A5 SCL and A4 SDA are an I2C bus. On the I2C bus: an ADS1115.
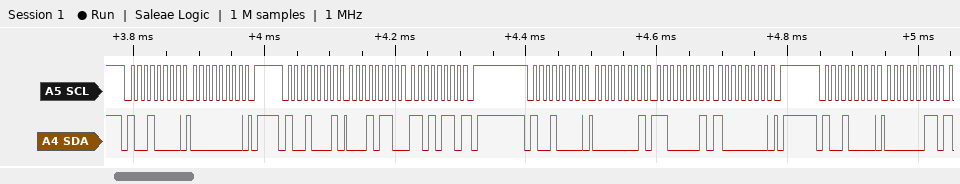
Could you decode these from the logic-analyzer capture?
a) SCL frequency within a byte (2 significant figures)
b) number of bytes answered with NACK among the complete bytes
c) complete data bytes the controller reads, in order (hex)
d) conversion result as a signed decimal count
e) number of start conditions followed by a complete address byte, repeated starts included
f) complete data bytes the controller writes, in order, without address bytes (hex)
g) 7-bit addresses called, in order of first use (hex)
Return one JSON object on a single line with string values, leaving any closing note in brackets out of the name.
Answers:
{"SCL frequency within a byte": "100 kHz", "number of bytes answered with NACK among the complete bytes": "1", "complete data bytes the controller reads, in order": "16 D6", "conversion result as a signed decimal count": "5846", "number of start conditions followed by a complete address byte, repeated starts included": "4", "complete data bytes the controller writes, in order, without address bytes": "00 01 C1 80 03", "7-bit addresses called, in order of first use": "0x48"}
